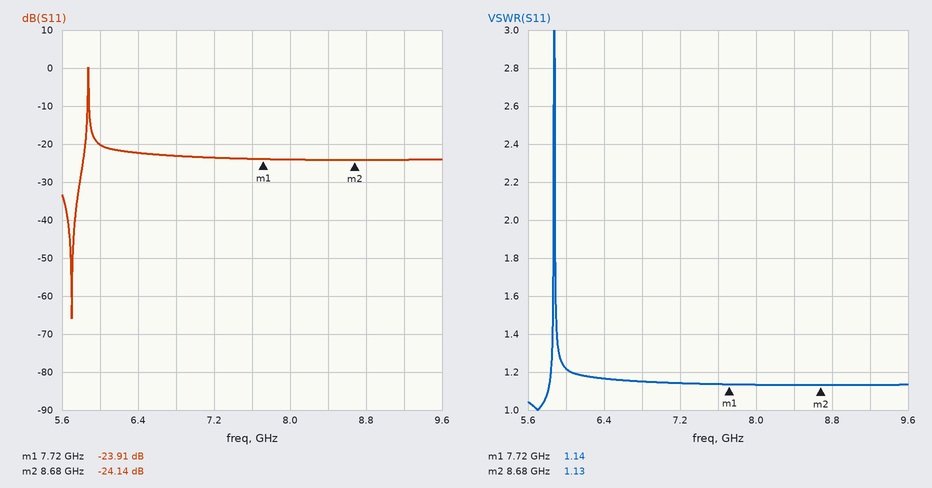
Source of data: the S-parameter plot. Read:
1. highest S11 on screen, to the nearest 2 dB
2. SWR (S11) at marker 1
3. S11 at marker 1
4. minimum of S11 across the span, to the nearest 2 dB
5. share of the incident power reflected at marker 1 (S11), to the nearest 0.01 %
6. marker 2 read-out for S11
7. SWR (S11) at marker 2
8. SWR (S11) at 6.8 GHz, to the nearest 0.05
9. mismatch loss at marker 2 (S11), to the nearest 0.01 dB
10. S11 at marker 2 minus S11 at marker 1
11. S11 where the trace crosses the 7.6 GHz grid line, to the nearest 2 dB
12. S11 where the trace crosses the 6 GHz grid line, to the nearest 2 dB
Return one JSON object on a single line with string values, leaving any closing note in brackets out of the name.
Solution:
{"highest S11 on screen, to the nearest 2 dB": "0 dB", "SWR (S11) at marker 1": "1.14", "S11 at marker 1": "-23.91 dB", "minimum of S11 across the span, to the nearest 2 dB": "-66 dB", "share of the incident power reflected at marker 1 (S11), to the nearest 0.01 %": "0.41 %", "marker 2 read-out for S11": "-24.14 dB", "SWR (S11) at marker 2": "1.13", "SWR (S11) at 6.8 GHz, to the nearest 0.05": "1.15", "mismatch loss at marker 2 (S11), to the nearest 0.01 dB": "0.02 dB", "S11 at marker 2 minus S11 at marker 1": "-0.23 dB", "S11 where the trace crosses the 7.6 GHz grid line, to the nearest 2 dB": "-24 dB", "S11 where the trace crosses the 6 GHz grid line, to the nearest 2 dB": "-20 dB"}
